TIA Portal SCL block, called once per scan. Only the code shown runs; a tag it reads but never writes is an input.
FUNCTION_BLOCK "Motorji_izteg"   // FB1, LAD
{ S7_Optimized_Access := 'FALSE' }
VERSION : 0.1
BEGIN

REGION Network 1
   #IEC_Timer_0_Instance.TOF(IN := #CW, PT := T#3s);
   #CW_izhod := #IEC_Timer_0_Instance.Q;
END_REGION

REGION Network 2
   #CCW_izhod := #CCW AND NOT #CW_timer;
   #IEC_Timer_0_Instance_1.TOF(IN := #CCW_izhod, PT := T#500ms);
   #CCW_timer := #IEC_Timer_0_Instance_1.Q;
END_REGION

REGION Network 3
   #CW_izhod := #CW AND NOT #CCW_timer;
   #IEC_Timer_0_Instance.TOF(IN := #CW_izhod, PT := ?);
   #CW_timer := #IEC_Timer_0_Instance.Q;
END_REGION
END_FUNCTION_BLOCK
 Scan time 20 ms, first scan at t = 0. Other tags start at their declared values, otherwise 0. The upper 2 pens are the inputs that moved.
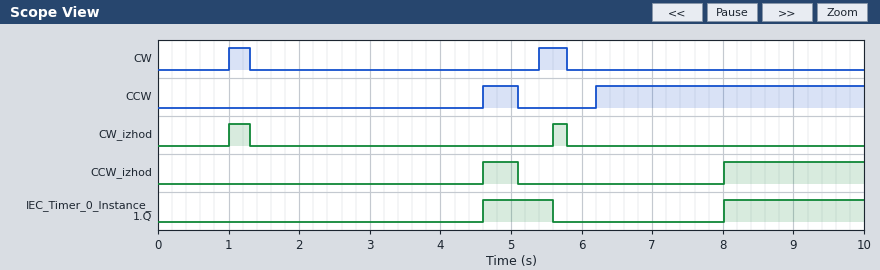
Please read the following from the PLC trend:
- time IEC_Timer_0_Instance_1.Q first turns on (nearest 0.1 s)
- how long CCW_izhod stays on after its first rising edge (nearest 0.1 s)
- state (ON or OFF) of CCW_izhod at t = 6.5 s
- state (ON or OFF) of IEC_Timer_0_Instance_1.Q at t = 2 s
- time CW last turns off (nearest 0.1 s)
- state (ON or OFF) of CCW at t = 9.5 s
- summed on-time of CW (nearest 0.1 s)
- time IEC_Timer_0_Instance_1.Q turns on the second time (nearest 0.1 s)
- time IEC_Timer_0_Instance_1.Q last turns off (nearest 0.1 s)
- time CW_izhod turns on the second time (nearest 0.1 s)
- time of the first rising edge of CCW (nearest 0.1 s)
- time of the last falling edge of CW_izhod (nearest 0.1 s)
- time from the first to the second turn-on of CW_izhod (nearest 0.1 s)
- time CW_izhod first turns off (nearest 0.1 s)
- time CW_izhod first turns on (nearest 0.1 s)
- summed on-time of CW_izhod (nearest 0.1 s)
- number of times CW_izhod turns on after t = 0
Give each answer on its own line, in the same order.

4.6 s
0.5 s
OFF
OFF
5.8 s
ON
0.7 s
8.0 s
5.6 s
5.6 s
4.6 s
5.8 s
4.6 s
1.3 s
1.0 s
0.5 s
2
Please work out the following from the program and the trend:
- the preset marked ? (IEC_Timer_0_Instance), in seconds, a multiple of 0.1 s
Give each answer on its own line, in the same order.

2.2 s
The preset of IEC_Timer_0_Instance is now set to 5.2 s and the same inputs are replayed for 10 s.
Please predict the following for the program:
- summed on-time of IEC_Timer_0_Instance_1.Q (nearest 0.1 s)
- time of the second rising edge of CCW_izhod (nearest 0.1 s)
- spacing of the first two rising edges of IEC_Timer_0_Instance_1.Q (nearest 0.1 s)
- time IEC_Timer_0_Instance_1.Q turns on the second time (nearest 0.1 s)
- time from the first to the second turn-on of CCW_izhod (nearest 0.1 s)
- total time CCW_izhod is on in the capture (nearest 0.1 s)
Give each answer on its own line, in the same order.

2.2 s
8.8 s
4.2 s
8.8 s
4.2 s
1.7 s
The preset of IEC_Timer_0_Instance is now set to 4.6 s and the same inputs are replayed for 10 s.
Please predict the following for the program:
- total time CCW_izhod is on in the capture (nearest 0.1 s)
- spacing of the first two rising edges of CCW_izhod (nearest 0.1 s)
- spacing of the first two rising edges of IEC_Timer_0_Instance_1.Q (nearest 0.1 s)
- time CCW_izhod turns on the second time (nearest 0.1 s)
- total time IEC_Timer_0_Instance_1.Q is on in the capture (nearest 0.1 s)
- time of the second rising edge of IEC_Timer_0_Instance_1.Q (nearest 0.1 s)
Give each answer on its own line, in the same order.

1.7 s
4.2 s
4.2 s
8.8 s
2.2 s
8.8 s
